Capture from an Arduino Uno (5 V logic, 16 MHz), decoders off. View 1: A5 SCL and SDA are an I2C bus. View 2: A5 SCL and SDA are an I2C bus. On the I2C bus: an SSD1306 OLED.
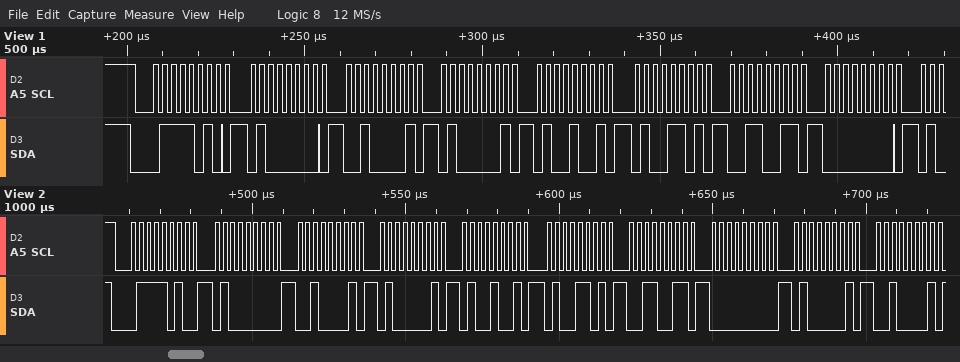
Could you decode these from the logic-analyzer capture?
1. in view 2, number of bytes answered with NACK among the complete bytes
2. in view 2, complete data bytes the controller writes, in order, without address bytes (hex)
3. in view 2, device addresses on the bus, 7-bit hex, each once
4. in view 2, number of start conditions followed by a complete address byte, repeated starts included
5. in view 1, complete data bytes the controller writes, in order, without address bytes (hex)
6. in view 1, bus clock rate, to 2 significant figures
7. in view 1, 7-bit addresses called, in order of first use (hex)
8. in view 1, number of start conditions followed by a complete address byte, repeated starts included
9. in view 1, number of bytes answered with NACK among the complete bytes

0
40 21 41 49 4D 33 00 41 21
0x3D
1
40 21 41 49 4D 33 00
400 kHz
0x3D
1
0
